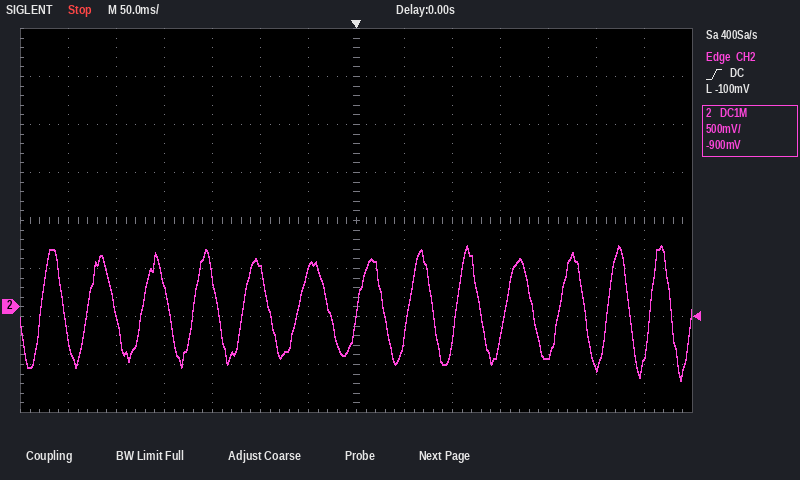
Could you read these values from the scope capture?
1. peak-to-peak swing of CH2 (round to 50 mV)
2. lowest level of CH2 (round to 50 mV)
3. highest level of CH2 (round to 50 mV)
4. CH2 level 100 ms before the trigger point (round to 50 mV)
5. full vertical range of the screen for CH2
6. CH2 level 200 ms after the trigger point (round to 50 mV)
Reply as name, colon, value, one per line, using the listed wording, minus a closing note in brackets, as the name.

peak-to-peak swing of CH2: 1.40 V
lowest level of CH2: -750 mV
highest level of CH2: 650 mV
CH2 level 100 ms before the trigger point: 400 mV
full vertical range of the screen for CH2: 4 V
CH2 level 200 ms after the trigger point: -500 mV
